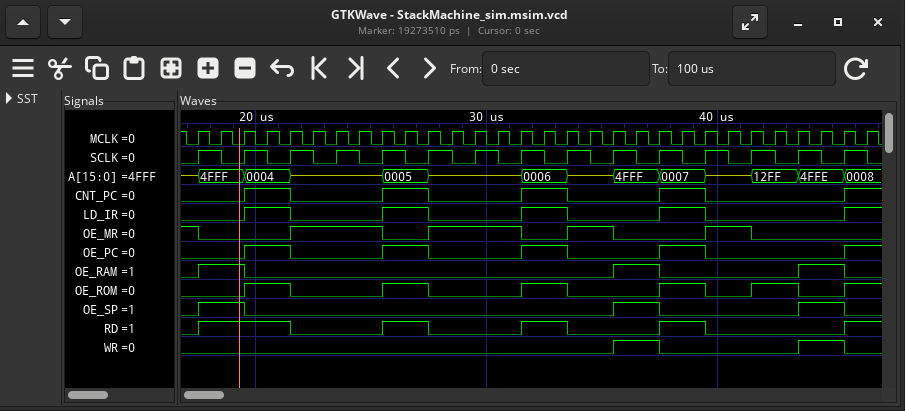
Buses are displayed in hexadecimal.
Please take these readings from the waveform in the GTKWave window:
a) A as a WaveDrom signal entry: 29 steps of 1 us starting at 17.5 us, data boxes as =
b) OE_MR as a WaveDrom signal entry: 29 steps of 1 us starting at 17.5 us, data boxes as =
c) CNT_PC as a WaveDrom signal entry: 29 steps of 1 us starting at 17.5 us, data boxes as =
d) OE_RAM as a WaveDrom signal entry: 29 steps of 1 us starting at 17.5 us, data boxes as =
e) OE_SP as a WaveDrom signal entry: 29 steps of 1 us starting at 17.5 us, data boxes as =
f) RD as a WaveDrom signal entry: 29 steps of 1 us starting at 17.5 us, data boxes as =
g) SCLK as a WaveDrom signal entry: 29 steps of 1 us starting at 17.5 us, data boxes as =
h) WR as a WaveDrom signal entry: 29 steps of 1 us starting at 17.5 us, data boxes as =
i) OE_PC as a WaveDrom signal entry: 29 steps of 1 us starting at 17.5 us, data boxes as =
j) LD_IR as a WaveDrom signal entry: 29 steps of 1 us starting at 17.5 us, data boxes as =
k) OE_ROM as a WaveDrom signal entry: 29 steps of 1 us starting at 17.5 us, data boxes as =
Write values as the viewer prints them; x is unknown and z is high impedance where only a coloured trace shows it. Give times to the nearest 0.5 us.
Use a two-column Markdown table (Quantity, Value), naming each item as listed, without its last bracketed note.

| Quantity | Value |
|---|---|
| A as a WaveDrom signal entry: 29 steps of 1 us starting at 17.5 us, data boxes as = | {name: 'A', wave: '=.=.z...=.z...=.z.=.=.z.=.=.=', data: '4FFF 0004 0005 0006 4FFF 0007 12FF 4FFE 0008'} |
| OE_MR as a WaveDrom signal entry: 29 steps of 1 us starting at 17.5 us, data boxes as = | {name: 'OE_MR', wave: '0...1...0.1...0.1.0...1.0....'} |
| CNT_PC as a WaveDrom signal entry: 29 steps of 1 us starting at 17.5 us, data boxes as = | {name: 'CNT_PC', wave: '0.1.0...1.0...1.0...1.0.....1'} |
| OE_RAM as a WaveDrom signal entry: 29 steps of 1 us starting at 17.5 us, data boxes as = | {name: 'OE_RAM', wave: '1.0...............1.0.....1.0'} |
| OE_SP as a WaveDrom signal entry: 29 steps of 1 us starting at 17.5 us, data boxes as = | {name: 'OE_SP', wave: '1.0...............1.0.....1.0'} |
| RD as a WaveDrom signal entry: 29 steps of 1 us starting at 17.5 us, data boxes as = | {name: 'RD', wave: '1...0...1.0...1.0...1.0.....1'} |
| SCLK as a WaveDrom signal entry: 29 steps of 1 us starting at 17.5 us, data boxes as = | {name: 'SCLK', wave: '10101010101010101010101010101'} |
| WR as a WaveDrom signal entry: 29 steps of 1 us starting at 17.5 us, data boxes as = | {name: 'WR', wave: '0.................1.0.....1.0'} |
| OE_PC as a WaveDrom signal entry: 29 steps of 1 us starting at 17.5 us, data boxes as = | {name: 'OE_PC', wave: '0.1.0...1.0...1.0...1.0.....1'} |
| LD_IR as a WaveDrom signal entry: 29 steps of 1 us starting at 17.5 us, data boxes as = | {name: 'LD_IR', wave: '0.1.0...1.0...1.0...1.0.....1'} |
| OE_ROM as a WaveDrom signal entry: 29 steps of 1 us starting at 17.5 us, data boxes as = | {name: 'OE_ROM', wave: '0.1.0...1.0...1.0...1.0.1.0.1'} |
